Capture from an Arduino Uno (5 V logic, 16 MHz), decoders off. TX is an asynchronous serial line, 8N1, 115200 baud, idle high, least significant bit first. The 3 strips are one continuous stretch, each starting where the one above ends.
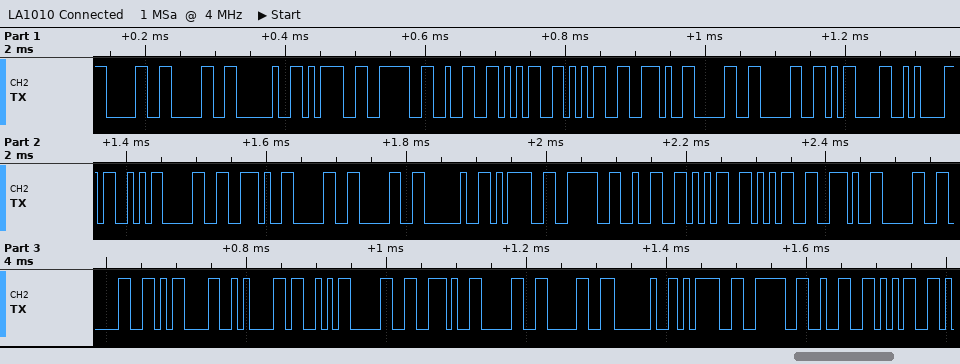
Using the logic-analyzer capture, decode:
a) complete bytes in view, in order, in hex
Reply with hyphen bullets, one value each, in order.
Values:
- 30 30 20 3D 3E 32 35 35 2E 30 30 0D 0A 53 30 2E 30 30 20 3D 3E 32 35 35 2E 30 30 0D 0A 53 30 2E 30 30 20 3D 3E 32 35
